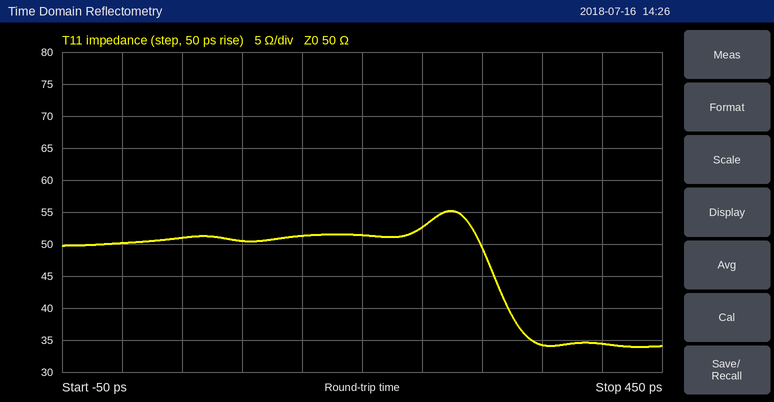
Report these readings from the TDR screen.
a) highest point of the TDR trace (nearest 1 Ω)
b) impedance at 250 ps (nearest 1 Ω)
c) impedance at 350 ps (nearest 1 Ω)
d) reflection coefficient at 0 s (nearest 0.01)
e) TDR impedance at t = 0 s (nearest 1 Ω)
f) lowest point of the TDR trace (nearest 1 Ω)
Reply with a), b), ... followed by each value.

a) 55 Ω
b) 53 Ω
c) 34 Ω
d) 0.00
e) 50 Ω
f) 34 Ω
